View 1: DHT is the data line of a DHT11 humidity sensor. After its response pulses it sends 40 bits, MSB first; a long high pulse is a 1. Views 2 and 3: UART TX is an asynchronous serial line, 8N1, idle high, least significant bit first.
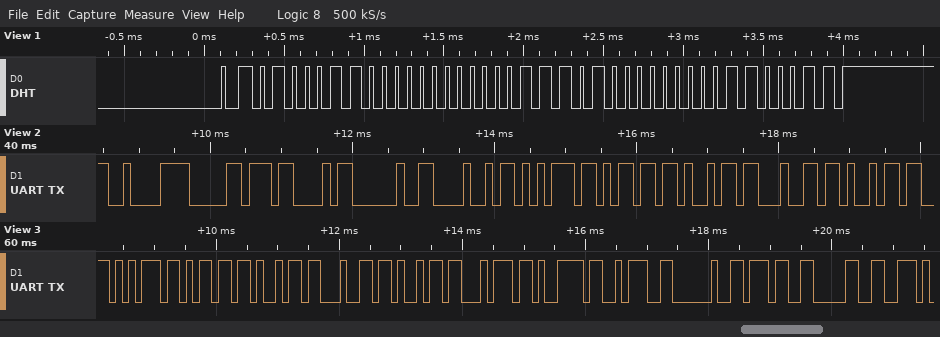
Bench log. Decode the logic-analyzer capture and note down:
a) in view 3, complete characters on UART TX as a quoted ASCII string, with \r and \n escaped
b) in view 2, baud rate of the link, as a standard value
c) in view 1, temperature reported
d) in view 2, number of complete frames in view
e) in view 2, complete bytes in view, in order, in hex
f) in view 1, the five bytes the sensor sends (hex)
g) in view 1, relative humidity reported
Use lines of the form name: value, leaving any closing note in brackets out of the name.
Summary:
in view 3, complete characters on UART TX as a quoted ASCII string, with \r and \n escaped: "umidity: 70"
in view 2, baud rate of the link, as a standard value: 9600 baud
in view 1, temperature reported: 29.0 °C
in view 2, number of complete frames in view: 10
in view 2, complete bytes in view, in order, in hex: C2 B0 43 20 48 75 6D 69 64 69
in view 1, the five bytes the sensor sends: 46 00 1D 00 63
in view 1, relative humidity reported: 70 %
